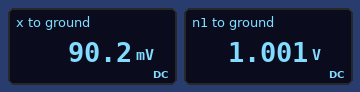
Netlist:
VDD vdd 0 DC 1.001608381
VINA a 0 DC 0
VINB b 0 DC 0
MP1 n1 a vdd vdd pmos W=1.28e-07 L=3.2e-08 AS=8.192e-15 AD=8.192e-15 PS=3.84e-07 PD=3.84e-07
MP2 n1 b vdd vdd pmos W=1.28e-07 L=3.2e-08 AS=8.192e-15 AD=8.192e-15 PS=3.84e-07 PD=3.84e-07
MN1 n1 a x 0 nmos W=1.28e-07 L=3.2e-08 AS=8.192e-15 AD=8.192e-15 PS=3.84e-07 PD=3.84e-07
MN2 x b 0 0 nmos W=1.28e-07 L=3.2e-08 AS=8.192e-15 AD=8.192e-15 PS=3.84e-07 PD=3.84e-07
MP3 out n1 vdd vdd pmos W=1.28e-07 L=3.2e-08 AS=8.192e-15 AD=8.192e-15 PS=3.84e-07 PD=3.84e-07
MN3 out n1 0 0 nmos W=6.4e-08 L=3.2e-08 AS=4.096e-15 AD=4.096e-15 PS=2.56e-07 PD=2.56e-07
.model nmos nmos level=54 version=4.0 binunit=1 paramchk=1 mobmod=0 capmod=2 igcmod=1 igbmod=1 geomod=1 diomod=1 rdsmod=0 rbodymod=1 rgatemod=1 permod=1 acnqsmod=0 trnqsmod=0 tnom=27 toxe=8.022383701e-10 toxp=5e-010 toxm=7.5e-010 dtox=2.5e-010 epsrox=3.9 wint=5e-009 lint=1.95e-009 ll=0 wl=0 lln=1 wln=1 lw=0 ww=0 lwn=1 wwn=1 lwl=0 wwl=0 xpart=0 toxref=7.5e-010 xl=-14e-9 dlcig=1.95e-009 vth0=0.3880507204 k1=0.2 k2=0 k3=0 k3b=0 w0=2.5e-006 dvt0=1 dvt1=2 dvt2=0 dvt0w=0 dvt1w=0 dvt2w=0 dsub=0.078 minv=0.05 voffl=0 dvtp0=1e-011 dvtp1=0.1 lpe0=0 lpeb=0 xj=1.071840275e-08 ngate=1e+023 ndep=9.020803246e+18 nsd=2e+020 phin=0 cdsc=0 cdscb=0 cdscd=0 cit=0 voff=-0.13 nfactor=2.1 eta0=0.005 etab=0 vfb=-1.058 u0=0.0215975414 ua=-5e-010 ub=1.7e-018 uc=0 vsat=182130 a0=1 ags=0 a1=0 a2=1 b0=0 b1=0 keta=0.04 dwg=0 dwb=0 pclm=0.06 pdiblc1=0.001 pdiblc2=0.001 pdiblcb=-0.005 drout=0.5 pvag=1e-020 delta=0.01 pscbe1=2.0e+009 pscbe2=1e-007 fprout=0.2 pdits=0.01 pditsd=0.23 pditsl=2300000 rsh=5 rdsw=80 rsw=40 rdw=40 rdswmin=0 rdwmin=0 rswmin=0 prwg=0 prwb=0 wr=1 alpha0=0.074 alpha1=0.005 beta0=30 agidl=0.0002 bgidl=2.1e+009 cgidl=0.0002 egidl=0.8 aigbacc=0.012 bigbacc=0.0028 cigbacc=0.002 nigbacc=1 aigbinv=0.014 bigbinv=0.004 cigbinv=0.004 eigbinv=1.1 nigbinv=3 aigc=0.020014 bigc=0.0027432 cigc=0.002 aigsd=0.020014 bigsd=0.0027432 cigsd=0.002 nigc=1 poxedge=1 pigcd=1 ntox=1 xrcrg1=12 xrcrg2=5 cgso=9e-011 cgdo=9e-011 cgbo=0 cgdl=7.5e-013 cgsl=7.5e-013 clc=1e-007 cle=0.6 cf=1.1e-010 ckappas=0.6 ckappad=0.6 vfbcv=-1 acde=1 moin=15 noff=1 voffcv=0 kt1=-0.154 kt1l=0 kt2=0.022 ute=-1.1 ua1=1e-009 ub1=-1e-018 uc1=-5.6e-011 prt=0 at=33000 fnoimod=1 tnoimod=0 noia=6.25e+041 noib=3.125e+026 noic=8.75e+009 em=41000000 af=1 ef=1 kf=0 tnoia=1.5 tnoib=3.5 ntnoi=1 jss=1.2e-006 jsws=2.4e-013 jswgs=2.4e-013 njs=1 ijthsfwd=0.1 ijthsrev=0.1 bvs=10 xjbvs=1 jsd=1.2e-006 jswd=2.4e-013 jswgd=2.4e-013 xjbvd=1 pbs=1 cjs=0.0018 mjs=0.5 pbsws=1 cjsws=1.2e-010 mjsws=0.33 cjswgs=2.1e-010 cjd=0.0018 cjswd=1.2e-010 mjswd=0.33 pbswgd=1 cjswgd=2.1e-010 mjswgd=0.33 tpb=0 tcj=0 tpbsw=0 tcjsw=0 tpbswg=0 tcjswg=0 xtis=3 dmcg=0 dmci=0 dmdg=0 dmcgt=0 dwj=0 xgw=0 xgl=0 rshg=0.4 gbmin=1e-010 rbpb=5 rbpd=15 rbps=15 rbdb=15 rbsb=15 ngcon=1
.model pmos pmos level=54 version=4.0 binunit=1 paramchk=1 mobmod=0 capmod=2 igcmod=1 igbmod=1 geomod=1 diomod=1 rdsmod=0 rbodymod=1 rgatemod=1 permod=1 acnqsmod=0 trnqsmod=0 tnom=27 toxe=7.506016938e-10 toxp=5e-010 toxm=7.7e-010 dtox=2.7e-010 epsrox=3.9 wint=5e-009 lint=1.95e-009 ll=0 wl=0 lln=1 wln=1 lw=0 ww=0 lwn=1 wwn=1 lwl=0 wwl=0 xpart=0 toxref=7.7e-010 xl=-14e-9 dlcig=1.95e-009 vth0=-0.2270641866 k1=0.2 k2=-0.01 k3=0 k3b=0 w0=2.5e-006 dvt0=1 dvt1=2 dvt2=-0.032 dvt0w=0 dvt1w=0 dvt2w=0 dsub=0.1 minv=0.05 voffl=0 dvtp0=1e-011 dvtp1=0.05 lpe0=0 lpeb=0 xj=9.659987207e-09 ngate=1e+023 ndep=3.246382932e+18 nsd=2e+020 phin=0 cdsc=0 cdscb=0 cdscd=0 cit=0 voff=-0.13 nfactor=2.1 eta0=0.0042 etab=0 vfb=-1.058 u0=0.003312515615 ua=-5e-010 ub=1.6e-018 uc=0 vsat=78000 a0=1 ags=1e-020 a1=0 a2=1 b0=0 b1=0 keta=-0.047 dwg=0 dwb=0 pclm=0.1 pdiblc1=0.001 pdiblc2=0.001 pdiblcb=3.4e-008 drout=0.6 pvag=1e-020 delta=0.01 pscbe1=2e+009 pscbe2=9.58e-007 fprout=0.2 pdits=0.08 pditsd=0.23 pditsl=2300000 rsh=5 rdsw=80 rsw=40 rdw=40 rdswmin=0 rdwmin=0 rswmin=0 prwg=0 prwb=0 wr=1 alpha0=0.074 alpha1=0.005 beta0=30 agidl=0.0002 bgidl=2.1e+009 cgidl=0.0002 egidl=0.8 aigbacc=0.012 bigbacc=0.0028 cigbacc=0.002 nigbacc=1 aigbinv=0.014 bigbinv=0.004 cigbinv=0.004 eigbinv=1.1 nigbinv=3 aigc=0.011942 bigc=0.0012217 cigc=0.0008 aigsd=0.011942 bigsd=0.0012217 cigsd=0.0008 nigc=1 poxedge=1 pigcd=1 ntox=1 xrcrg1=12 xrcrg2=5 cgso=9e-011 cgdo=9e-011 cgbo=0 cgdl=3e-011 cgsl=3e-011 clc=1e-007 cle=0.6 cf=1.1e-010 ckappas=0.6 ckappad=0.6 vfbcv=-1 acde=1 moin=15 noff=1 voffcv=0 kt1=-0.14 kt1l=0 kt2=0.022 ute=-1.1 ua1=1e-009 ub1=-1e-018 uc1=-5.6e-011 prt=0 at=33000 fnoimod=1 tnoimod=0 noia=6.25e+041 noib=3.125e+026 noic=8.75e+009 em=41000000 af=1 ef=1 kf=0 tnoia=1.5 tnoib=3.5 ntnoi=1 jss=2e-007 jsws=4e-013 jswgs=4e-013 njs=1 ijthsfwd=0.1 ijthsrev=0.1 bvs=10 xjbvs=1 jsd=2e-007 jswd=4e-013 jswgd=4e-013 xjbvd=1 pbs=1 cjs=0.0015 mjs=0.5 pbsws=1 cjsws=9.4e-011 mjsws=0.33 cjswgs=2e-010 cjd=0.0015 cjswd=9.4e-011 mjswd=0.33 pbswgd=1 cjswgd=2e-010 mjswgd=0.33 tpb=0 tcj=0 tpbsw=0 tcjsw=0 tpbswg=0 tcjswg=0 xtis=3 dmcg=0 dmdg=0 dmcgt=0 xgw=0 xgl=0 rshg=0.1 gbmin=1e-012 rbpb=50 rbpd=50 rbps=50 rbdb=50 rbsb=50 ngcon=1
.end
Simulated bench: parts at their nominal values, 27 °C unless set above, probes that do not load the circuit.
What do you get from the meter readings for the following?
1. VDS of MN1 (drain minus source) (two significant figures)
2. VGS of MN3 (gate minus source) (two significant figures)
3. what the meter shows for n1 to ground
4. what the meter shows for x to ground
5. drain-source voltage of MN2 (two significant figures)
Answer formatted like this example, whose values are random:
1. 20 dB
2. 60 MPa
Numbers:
1. 910 mV
2. 1.0 V
3. 1.001 V
4. 90.2 mV
5. 90 mV
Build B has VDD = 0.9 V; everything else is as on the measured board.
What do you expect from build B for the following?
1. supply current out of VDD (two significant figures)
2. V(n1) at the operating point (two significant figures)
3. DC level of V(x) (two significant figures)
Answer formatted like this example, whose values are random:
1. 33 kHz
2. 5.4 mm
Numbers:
1. 220 nA
2. 900 mV
3. 81 mV
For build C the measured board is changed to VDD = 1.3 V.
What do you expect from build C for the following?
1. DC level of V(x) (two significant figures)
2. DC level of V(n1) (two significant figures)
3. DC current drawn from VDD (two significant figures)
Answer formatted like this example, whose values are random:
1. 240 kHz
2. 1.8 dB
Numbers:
1. 120 mV
2. 1.3 V
3. 2.0 µA
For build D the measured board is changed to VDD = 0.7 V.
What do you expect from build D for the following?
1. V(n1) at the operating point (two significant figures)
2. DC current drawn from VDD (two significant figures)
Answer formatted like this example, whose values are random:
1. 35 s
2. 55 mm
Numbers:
1. 700 mV
2. 110 nA
